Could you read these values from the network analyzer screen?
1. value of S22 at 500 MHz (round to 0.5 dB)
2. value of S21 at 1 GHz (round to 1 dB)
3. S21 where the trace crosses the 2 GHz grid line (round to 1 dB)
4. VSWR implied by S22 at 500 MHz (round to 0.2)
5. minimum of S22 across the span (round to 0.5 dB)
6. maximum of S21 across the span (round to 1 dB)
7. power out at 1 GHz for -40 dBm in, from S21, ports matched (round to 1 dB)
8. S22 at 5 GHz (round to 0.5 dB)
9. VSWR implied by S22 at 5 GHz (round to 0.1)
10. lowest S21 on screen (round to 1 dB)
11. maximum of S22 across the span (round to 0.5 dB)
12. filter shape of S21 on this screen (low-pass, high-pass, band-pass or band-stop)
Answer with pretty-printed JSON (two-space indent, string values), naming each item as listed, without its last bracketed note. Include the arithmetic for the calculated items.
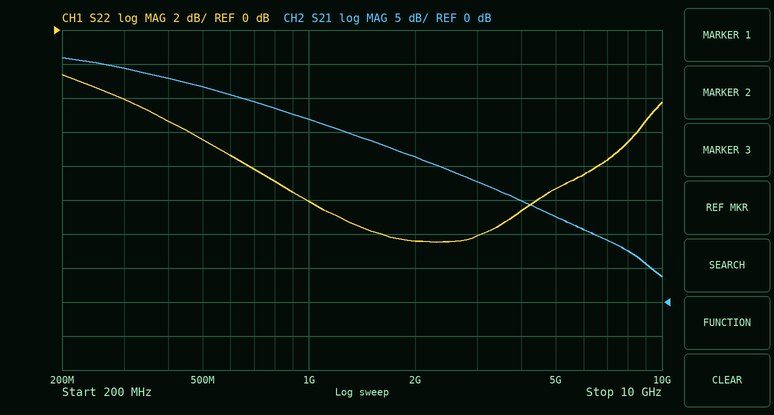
{
  "value of S22 at 500 MHz": "-6.5 dB",
  "value of S21 at 1 GHz": "27 dB",
  "S21 where the trace crosses the 2 GHz grid line": "21 dB",
  "VSWR implied by S22 at 500 MHz": "|Γ| = 10^(-6.5/20) = 0.4732; VSWR = (1 + 0.4732)/(1 − 0.4732) ≈ 2.8",
  "minimum of S22 across the span": "-12.5 dB",
  "maximum of S21 across the span": "36 dB",
  "power out at 1 GHz for -40 dBm in, from S21, ports matched": "-40 dBm + (27 dB) = -13 dBm",
  "S22 at 5 GHz": "-9.5 dB",
  "VSWR implied by S22 at 5 GHz": "|Γ| = 10^(-9.5/20) = 0.3350; VSWR = (1 + 0.3350)/(1 − 0.3350) ≈ 2.0",
  "lowest S21 on screen": "4 dB",
  "maximum of S22 across the span": "-2.5 dB",
  "filter shape of S21 on this screen": "low-pass"
}
